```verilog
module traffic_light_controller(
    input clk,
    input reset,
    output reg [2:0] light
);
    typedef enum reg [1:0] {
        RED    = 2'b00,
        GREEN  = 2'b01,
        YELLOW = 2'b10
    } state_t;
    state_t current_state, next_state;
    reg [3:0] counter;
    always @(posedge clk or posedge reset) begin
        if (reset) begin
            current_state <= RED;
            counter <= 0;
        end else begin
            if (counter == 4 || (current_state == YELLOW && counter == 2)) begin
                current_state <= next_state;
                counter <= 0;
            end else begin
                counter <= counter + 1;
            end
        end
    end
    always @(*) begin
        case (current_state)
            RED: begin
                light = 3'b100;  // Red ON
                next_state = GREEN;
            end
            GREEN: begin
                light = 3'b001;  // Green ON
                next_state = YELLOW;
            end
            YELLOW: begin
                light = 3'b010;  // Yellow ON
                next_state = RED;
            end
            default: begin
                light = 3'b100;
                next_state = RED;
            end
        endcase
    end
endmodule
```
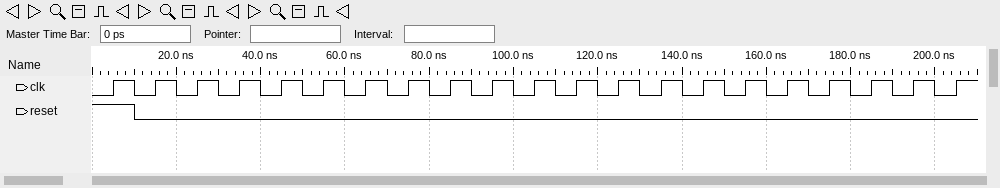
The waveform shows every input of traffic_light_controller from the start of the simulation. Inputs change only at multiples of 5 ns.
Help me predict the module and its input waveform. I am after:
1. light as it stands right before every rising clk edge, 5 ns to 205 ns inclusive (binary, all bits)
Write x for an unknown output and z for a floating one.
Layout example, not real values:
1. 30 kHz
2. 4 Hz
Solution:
1. 100, 100, 100, 100, 100, 100, 001, 001, 001, 001, 001, 010, 010, 010, 100, 100, 100, 100, 100, 001, 001
